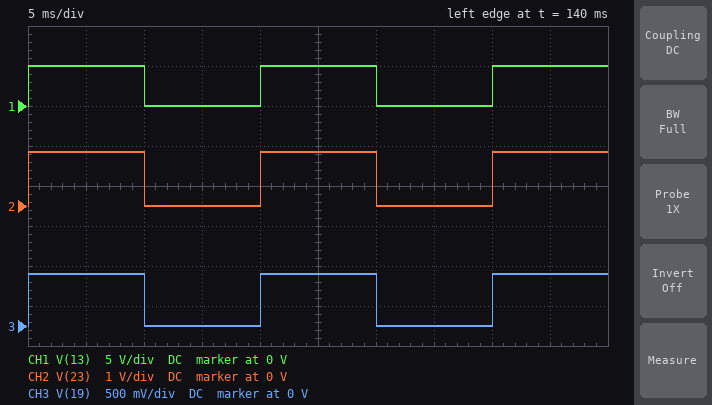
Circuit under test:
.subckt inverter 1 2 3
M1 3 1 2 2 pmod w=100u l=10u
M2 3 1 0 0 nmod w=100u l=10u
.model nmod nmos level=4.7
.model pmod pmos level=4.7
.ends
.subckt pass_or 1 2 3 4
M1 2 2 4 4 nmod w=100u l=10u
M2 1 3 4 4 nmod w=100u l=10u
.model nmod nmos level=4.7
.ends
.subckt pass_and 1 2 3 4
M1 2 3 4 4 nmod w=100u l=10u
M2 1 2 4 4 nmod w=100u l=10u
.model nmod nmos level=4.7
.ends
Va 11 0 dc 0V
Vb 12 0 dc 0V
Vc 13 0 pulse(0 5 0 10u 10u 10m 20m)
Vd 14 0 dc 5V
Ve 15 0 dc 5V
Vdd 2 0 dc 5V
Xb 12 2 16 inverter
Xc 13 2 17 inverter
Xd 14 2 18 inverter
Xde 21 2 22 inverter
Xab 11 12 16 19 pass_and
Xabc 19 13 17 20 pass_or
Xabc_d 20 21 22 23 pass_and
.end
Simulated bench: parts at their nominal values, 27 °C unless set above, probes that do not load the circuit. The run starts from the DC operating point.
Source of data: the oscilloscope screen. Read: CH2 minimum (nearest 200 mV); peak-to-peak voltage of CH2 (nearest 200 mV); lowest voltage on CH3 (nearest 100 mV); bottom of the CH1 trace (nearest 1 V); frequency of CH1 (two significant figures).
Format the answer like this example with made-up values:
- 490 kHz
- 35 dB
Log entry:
- 0 V
- 1.4 V
- 0 V
- 0 V
- 50 Hz
